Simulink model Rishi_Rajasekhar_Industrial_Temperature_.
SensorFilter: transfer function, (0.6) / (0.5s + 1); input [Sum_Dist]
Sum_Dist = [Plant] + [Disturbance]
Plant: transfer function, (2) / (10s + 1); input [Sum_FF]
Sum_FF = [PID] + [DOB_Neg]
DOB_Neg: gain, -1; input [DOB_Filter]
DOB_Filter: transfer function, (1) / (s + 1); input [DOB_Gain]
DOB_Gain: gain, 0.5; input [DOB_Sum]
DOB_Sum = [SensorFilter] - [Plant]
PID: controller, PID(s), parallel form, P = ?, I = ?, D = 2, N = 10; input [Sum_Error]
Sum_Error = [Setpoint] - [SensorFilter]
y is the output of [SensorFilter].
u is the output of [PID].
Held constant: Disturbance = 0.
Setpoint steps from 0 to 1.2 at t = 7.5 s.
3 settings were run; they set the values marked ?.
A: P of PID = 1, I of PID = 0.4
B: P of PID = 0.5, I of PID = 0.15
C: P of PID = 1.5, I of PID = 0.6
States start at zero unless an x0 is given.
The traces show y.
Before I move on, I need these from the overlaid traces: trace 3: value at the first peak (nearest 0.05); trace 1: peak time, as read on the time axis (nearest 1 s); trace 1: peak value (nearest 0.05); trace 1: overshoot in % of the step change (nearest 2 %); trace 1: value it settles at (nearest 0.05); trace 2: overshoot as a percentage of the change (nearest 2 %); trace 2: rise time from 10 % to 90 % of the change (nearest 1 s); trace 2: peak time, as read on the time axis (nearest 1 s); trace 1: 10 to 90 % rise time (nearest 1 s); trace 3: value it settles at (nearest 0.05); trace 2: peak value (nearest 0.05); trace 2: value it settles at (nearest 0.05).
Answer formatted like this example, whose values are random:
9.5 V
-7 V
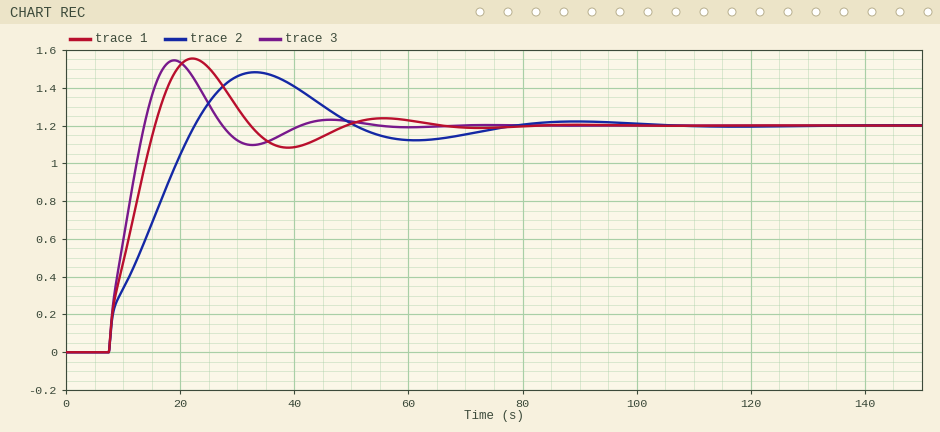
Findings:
1.55
22 s
1.55
30 %
1.20
24 %
13 s
33 s
7 s
1.20
1.50
1.20
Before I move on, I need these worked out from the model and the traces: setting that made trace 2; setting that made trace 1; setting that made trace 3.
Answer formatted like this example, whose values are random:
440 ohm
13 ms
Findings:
B
A
C
